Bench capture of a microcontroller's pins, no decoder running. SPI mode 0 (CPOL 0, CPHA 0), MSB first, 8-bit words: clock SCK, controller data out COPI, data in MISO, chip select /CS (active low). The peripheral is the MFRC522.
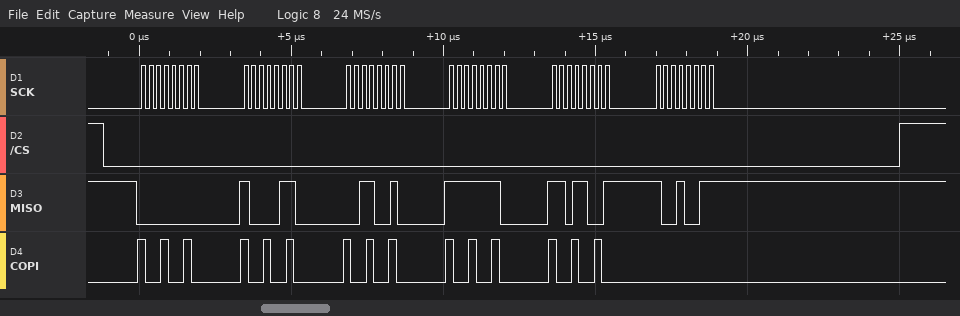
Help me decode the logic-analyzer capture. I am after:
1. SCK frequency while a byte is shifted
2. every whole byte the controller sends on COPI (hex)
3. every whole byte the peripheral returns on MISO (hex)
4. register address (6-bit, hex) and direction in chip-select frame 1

4 MHz
92 92 92 92 92 00
00 86 32 FE D9 93
0x09 read
